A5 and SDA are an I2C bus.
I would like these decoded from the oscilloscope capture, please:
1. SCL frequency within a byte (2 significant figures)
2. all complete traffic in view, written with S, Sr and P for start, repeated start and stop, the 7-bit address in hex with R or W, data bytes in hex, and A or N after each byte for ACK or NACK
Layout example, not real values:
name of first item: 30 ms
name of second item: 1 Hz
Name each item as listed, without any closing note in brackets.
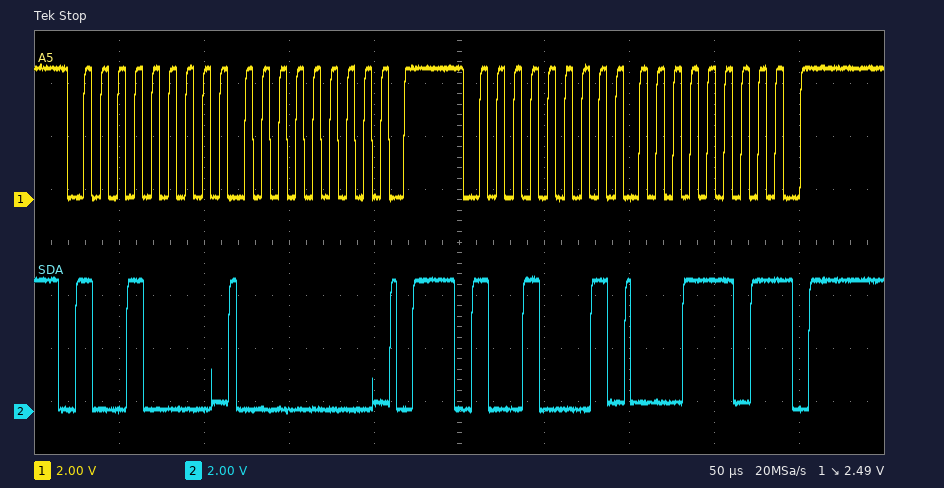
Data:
SCL frequency within a byte: 100 kHz
all complete traffic in view, written with S, Sr and P for start, repeated start and stop, the 7-bit address in hex with R or W, data bytes in hex, and A or N after each byte for ACK or NACK: S 48W A 00 A P S 48R A 1D N P
